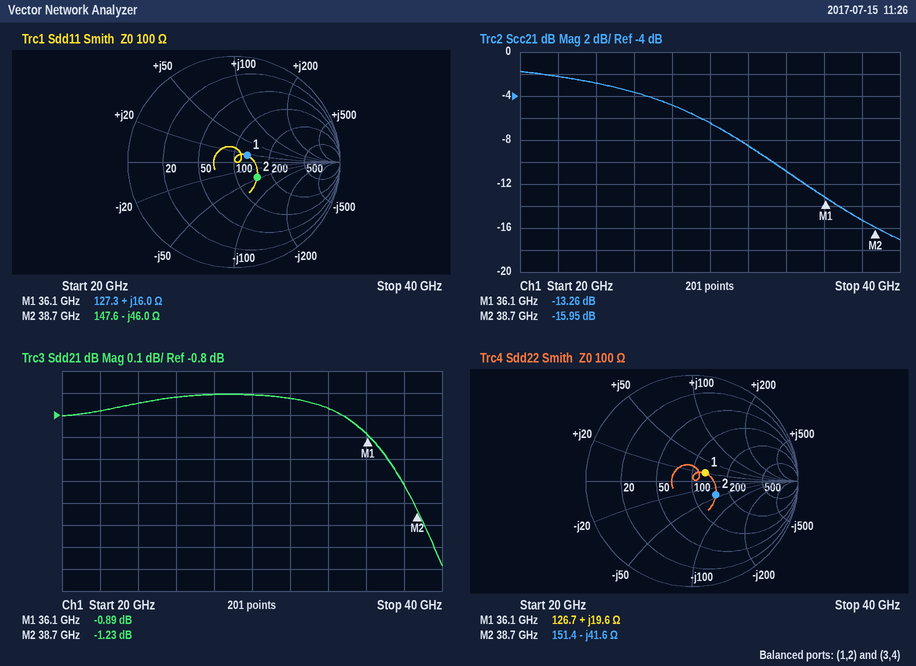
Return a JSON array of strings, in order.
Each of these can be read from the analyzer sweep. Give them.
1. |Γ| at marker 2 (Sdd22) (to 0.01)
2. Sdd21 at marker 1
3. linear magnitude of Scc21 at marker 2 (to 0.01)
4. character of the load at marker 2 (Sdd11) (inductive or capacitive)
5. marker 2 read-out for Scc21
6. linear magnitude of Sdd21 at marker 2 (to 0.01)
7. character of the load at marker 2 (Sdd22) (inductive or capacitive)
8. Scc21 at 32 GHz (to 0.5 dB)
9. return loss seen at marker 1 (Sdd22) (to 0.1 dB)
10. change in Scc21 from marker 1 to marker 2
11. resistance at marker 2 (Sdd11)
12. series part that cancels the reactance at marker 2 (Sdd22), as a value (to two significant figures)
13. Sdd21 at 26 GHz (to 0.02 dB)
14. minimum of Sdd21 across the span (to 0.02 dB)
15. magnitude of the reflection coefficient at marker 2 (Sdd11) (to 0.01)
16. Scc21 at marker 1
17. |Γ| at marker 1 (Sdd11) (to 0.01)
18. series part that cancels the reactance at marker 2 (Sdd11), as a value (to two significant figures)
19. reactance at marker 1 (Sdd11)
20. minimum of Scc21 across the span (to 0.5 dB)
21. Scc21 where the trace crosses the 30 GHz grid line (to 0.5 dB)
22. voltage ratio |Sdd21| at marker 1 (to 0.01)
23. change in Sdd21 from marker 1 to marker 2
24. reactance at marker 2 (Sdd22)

["0.26", "-0.89 dB", "0.16", "capacitive", "-15.95 dB", "0.87", "capacitive", "-8.5 dB", "16.7 dB", "-2.69 dB", "147.6 Ω", "170 pH", "-0.72 dB", "-1.48 dB", "0.26", "-13.26 dB", "0.14", "190 pH", "+16.0 Ω", "-17.0 dB", "-6.5 dB", "0.90", "-0.34 dB", "-41.6 Ω"]
